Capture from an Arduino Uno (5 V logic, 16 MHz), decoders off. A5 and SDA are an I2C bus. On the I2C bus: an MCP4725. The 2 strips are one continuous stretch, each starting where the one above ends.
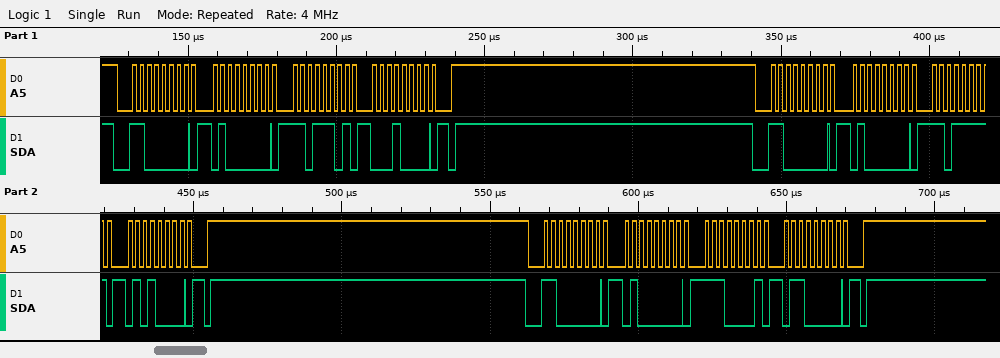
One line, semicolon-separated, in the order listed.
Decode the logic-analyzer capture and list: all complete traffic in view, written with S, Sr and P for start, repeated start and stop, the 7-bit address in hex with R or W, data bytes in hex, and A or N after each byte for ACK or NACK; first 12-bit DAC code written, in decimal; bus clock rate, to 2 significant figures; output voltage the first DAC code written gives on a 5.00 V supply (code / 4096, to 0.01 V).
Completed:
S 60W A 40 A DD A 10 A P S 60W A 40 A DF A 50 A P S 60W A 40 A E1 A 60 A P; 3537; 400 kHz; 4.32 V
